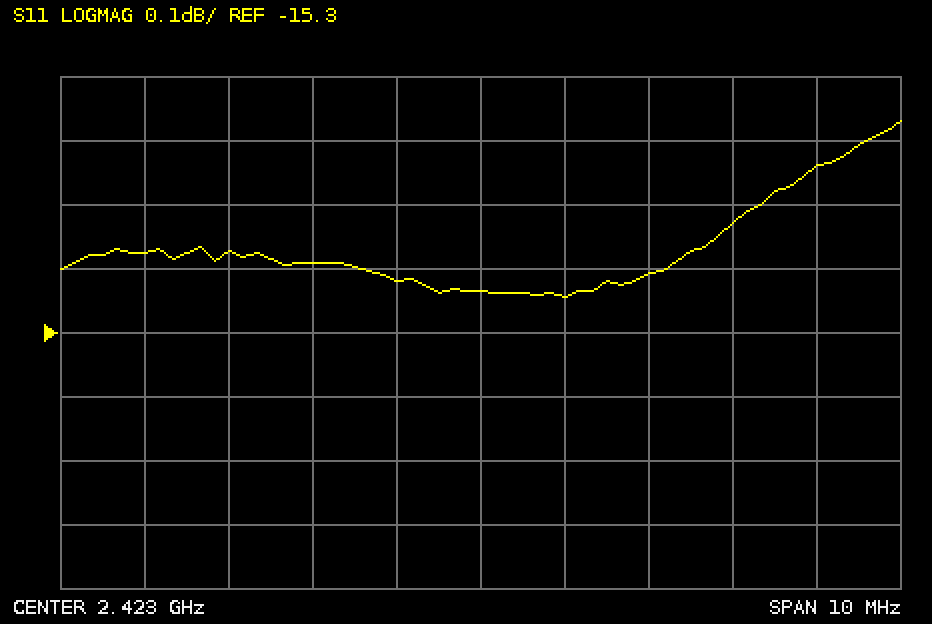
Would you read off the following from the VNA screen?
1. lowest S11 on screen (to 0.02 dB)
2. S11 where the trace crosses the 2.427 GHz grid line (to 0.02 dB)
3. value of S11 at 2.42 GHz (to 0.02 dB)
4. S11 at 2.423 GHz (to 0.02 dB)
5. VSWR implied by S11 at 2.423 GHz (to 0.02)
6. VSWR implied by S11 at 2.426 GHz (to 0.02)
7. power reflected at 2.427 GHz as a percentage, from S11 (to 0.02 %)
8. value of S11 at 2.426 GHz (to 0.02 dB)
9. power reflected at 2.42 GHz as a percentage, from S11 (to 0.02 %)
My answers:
-15.24 dB
-15.04 dB
-15.18 dB
-15.24 dB
1.42
1.42
3.14 %
-15.12 dB
3.04 %
